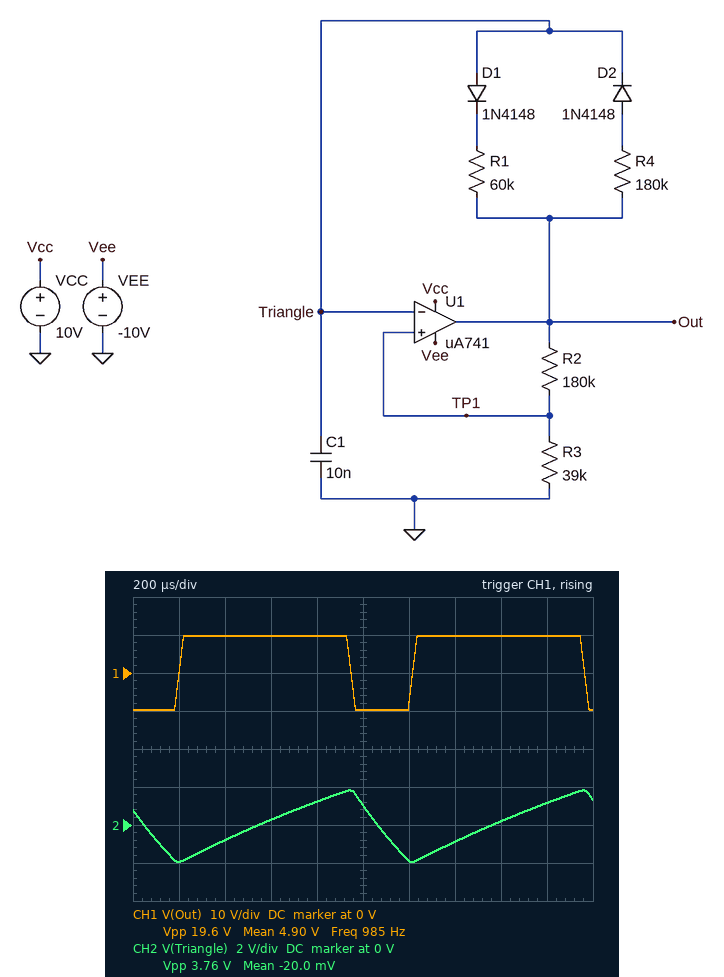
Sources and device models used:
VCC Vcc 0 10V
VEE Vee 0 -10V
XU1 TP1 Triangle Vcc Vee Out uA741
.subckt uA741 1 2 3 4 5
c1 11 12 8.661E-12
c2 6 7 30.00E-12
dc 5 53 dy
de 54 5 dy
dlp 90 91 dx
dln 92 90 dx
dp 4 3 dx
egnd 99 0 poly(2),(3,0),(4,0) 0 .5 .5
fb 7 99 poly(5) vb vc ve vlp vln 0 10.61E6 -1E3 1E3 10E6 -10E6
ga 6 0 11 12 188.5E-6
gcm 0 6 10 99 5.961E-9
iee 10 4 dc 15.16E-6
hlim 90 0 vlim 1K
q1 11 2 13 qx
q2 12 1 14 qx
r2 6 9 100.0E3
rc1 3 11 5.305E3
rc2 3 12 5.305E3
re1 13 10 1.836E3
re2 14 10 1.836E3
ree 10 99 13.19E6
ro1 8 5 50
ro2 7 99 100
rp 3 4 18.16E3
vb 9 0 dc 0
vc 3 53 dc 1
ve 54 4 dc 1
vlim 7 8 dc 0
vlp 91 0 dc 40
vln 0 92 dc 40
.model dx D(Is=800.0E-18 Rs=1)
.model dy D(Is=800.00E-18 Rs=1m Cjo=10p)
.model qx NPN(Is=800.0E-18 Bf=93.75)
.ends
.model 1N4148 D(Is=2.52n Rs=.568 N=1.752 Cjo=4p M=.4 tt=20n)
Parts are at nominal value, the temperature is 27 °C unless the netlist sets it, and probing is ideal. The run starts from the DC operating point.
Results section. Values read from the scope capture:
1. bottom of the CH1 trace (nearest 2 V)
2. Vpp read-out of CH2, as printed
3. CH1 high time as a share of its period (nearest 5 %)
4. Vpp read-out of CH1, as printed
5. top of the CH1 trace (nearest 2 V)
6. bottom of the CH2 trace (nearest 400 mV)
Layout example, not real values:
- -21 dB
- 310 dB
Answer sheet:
- -10 V
- 3.76 V
- 75 %
- 19.6 V
- 10 V
- -2.0 V
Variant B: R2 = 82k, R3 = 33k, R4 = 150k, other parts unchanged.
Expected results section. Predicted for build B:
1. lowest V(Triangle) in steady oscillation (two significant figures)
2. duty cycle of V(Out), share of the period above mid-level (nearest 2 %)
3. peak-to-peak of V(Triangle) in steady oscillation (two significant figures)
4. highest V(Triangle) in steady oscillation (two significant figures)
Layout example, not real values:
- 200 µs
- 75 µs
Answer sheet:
- -3.0 V
- 70 %
- 5.9 V
- 2.9 V
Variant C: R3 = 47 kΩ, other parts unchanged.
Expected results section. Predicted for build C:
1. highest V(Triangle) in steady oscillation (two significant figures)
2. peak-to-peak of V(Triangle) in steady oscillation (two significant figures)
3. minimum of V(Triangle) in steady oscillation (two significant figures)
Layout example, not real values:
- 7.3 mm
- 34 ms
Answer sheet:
- 2.1 V
- 4.3 V
- -2.2 V
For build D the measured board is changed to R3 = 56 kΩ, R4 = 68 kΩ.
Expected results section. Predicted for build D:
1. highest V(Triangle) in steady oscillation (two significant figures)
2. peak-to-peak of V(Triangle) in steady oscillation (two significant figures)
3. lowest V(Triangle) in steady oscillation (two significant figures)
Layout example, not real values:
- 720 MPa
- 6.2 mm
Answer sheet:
- 2.5 V
- 5.0 V
- -2.5 V
